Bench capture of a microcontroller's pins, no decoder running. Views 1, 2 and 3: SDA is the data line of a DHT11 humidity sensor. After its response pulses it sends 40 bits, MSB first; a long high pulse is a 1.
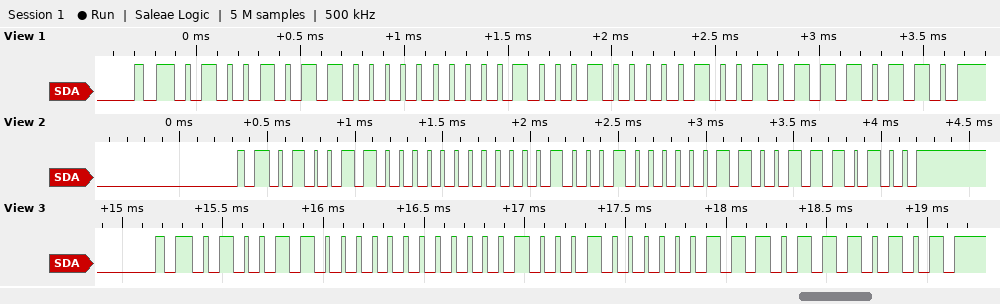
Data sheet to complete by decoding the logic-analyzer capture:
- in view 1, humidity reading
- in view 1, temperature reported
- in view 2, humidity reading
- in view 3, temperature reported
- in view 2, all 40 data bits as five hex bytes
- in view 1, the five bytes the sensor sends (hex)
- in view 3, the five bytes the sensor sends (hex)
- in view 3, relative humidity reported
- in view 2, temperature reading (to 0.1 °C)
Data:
75 %
34.9 °C
76 %
34.7 °C
4C 00 22 06 74
4B 00 22 09 76
4C 00 22 07 75
76 %
34.6 °C
